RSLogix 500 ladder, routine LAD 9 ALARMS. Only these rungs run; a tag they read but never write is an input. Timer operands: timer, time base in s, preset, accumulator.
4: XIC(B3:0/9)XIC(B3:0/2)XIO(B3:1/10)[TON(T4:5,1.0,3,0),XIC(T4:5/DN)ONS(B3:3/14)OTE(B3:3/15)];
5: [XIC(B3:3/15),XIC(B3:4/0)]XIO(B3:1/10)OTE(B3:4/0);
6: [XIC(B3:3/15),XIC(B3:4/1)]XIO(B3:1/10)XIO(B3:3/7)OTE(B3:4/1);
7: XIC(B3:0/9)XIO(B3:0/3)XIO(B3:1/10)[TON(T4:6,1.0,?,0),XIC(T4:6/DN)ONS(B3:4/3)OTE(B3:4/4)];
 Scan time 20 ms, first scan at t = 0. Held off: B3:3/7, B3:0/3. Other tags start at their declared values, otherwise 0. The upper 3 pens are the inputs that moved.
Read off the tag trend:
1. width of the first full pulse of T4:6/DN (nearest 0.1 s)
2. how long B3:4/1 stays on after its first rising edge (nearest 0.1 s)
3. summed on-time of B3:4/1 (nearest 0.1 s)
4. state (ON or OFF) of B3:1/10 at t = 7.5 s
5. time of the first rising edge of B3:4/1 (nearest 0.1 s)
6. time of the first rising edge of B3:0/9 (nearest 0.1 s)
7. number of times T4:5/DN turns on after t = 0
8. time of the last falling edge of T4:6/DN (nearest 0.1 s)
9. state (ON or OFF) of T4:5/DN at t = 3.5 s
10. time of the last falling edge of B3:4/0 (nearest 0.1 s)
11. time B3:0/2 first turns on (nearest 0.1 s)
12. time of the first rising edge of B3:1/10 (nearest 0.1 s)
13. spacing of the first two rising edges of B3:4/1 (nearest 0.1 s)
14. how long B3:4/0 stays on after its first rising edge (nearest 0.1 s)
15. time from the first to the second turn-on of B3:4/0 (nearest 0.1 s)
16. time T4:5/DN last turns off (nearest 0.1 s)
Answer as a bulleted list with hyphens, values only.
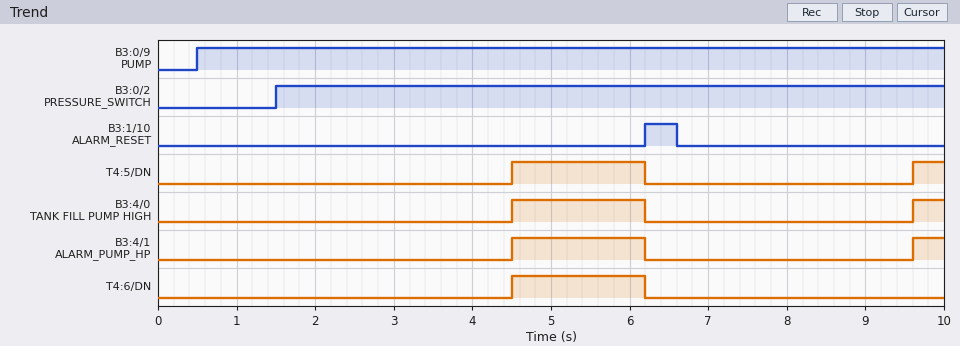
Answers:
- 1.7 s
- 1.7 s
- 2.1 s
- OFF
- 4.5 s
- 0.5 s
- 2
- 6.2 s
- OFF
- 6.2 s
- 1.5 s
- 6.2 s
- 5.1 s
- 1.7 s
- 5.1 s
- 6.2 s
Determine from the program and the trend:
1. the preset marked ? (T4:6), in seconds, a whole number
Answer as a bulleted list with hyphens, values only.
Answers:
- 4 s
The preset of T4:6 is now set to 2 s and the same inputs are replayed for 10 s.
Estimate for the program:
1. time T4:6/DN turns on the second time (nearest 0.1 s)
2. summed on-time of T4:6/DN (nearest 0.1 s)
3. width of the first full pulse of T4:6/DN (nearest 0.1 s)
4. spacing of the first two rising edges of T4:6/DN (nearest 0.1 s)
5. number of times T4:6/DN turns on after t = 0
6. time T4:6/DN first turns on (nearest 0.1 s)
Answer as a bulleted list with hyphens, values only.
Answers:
- 8.6 s
- 5.1 s
- 3.7 s
- 6.1 s
- 2
- 2.5 s
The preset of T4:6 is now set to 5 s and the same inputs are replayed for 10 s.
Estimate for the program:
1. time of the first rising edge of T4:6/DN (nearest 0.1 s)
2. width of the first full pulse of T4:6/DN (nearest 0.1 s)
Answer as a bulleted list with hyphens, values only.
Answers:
- 5.5 s
- 0.7 s
